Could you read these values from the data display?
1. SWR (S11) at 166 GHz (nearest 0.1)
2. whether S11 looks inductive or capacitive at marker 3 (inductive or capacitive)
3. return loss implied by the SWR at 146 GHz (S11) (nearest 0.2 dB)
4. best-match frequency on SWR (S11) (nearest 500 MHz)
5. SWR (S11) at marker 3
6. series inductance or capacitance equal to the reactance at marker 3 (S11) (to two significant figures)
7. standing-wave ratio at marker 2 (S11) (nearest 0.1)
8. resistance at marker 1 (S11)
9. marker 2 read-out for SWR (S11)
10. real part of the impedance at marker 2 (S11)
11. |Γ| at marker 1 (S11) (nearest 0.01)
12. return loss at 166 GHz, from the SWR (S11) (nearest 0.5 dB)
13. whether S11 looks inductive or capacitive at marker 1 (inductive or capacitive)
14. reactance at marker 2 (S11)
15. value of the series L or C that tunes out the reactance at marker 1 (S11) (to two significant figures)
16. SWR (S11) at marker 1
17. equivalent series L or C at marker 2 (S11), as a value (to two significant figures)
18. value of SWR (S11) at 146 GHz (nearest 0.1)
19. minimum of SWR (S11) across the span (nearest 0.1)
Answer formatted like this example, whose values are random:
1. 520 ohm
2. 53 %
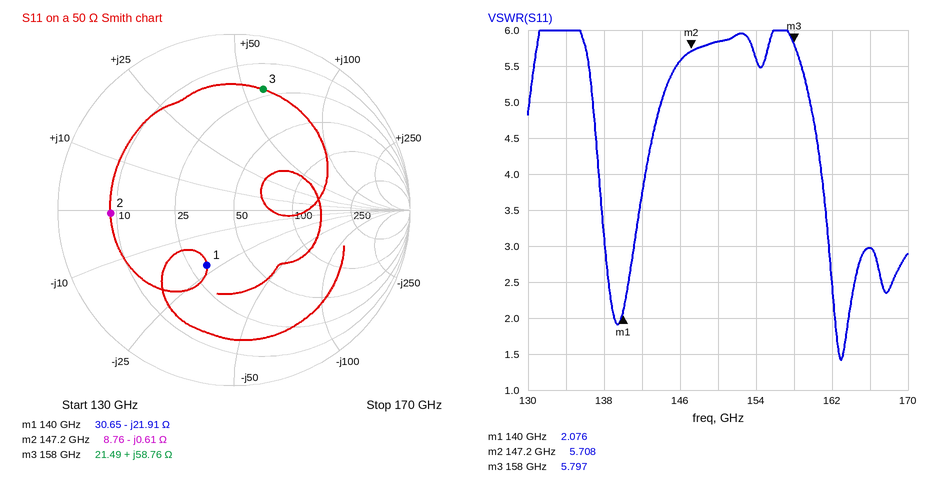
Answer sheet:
1. 3.0
2. inductive
3. 3.2 dB
4. 163.0 GHz
5. 5.797
6. 59 pH
7. 5.7
8. 30.65 Ω
9. 5.708
10. 8.76 Ω
11. 0.35
12. 6.0 dB
13. capacitive
14. -0.61 Ω
15. 25 pH
16. 2.076
17. 1.8 pF
18. 5.6
19. 1.4
